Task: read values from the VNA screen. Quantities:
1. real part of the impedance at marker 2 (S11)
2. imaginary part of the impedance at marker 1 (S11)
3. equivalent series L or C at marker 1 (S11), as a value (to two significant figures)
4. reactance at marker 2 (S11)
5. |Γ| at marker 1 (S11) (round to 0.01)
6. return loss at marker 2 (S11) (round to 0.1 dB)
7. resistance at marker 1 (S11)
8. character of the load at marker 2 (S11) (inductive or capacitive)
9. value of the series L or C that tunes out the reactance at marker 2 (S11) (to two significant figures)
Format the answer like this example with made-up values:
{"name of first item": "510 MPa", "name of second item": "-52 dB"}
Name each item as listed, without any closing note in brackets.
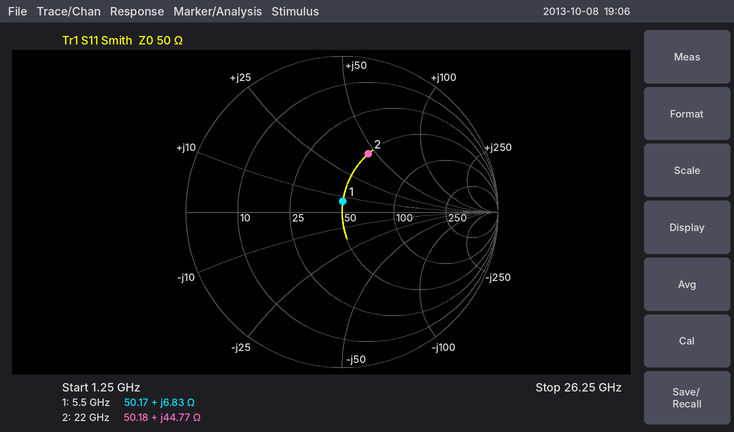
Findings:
{"real part of the impedance at marker 2": "50.18 Ω", "imaginary part of the impedance at marker 1": "+6.83 Ω", "equivalent series L or C at marker 1 (S11), as a value": "200 pH", "reactance at marker 2": "+44.77 Ω", "|Γ| at marker 1 (S11)": "0.07", "return loss at marker 2 (S11)": "7.8 dB", "resistance at marker 1": "50.17 Ω", "character of the load at marker 2 (S11)": "inductive", "value of the series L or C that tunes out the reactance at marker 2 (S11)": "160 fF"}
